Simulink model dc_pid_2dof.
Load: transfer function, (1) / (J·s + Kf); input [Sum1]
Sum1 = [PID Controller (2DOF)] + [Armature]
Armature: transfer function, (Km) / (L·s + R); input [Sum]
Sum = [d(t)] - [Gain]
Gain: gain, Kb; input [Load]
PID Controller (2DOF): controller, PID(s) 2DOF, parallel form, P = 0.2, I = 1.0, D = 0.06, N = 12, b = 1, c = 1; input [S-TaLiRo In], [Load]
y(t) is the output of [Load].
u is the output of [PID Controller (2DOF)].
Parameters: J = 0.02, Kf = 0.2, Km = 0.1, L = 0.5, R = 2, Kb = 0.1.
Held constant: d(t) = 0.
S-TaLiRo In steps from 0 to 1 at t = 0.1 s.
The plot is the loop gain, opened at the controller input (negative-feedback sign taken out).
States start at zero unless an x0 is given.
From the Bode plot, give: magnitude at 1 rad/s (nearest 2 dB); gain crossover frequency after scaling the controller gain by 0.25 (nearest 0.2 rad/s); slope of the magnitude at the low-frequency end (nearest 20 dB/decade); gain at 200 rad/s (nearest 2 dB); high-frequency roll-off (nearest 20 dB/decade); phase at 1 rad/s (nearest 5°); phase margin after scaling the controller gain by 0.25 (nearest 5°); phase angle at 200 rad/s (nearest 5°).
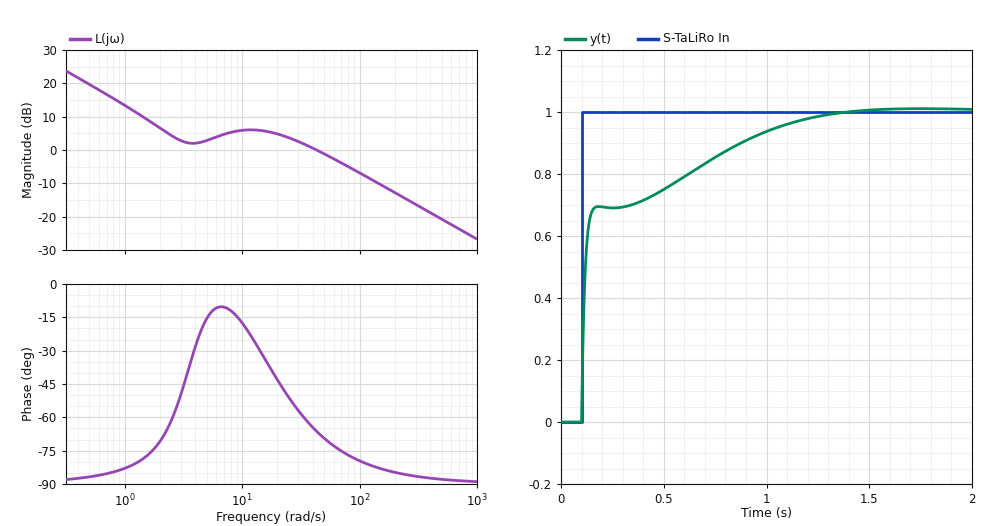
14 dB
1.2 rad/s
-20 dB/decade
-12 dB
-20 dB/decade
-85°
100°
-85°
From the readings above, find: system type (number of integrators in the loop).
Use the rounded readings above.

1
